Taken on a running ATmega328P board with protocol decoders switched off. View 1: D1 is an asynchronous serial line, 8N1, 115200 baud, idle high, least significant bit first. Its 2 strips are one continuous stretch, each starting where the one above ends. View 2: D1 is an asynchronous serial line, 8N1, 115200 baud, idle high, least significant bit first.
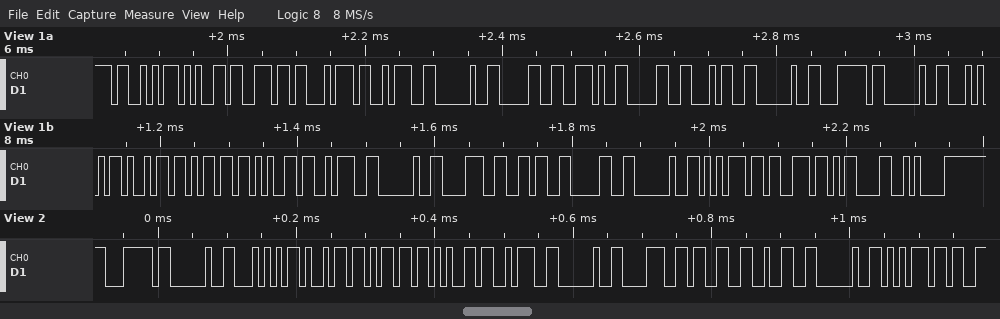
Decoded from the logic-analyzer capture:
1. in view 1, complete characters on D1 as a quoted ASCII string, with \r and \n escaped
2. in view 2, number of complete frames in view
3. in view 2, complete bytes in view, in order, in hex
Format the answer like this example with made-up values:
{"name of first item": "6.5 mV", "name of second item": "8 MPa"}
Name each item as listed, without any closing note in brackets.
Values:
{"in view 1, complete characters on D1 as a quoted ASCII string, with \\r and \\n escaped": "\"Sent: 0.04 | Time: 860 us\\r\\n\"", "in view 2, number of complete frames in view": "13", "in view 2, complete bytes in view, in order, in hex": "0x7C 0x20 0x54 0x69 0x6D 0x65 0x3A 0x20 0x38 0x33 0x32 0x20 0x75"}
